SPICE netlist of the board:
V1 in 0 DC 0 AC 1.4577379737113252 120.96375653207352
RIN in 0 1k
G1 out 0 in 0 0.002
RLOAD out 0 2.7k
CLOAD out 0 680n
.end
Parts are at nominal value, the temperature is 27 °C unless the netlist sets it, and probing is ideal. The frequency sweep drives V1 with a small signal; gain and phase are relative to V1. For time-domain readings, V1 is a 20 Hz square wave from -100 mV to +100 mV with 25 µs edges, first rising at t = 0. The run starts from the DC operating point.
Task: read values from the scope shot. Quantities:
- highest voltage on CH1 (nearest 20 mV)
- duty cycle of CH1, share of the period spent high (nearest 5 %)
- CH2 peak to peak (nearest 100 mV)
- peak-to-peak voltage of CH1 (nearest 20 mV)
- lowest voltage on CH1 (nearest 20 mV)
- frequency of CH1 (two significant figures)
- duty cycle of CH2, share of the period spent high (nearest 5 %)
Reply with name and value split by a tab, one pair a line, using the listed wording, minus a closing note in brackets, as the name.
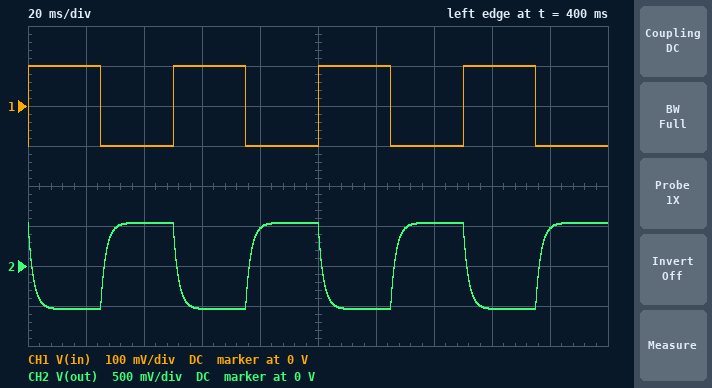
highest voltage on CH1	100 mV
duty cycle of CH1, share of the period spent high	50 %
CH2 peak to peak	1.1 V
peak-to-peak voltage of CH1	200 mV
lowest voltage on CH1	-100 mV
frequency of CH1	20 Hz
duty cycle of CH2, share of the period spent high	50 %
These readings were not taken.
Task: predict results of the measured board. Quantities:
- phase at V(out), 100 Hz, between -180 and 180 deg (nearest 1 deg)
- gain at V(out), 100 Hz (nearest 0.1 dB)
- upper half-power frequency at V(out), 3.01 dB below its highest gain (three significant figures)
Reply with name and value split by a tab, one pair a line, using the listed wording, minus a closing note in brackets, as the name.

phase at V(out), 100 Hz, between -180 and 180 deg	131 deg
gain at V(out), 100 Hz	11.0 dB
upper half-power frequency at V(out), 3.01 dB below its highest gain	86.7 Hz
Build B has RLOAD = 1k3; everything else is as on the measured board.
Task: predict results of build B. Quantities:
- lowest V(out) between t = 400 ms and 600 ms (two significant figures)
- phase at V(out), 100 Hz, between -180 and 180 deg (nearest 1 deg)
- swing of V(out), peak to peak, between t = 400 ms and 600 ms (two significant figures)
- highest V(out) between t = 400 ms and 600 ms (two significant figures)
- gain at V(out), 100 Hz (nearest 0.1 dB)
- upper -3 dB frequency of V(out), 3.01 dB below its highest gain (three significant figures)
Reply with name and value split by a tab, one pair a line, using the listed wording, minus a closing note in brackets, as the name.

lowest V(out) between t = 400 ms and 600 ms	-260 mV
phase at V(out), 100 Hz, between -180 and 180 deg	151 deg
swing of V(out), peak to peak, between t = 400 ms and 600 ms	520 mV
highest V(out) between t = 400 ms and 600 ms	260 mV
gain at V(out), 100 Hz	7.1 dB
upper -3 dB frequency of V(out), 3.01 dB below its highest gain	180 Hz
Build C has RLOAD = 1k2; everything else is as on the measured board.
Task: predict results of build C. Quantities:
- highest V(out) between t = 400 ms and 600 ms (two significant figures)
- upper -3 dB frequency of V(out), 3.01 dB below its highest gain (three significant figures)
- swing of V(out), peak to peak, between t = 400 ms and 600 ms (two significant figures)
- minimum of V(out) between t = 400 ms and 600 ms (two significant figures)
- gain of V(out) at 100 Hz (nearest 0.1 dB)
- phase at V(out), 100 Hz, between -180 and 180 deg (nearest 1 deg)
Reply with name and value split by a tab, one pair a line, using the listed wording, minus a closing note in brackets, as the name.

highest V(out) between t = 400 ms and 600 ms	240 mV
upper -3 dB frequency of V(out), 3.01 dB below its highest gain	195 Hz
swing of V(out), peak to peak, between t = 400 ms and 600 ms	480 mV
minimum of V(out) between t = 400 ms and 600 ms	-240 mV
gain of V(out) at 100 Hz	6.6 dB
phase at V(out), 100 Hz, between -180 and 180 deg	153 deg
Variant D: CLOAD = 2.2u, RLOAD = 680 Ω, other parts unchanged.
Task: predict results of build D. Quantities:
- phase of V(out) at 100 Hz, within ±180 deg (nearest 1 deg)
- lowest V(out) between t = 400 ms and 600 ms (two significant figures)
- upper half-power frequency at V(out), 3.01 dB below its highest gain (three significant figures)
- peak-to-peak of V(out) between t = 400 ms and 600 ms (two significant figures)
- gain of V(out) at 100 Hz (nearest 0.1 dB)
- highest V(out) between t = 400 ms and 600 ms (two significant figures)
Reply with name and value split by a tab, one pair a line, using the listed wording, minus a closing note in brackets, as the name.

phase of V(out) at 100 Hz, within ±180 deg	137 deg
lowest V(out) between t = 400 ms and 600 ms	-140 mV
upper half-power frequency at V(out), 3.01 dB below its highest gain	106 Hz
peak-to-peak of V(out) between t = 400 ms and 600 ms	270 mV
gain of V(out) at 100 Hz	-0.1 dB
highest V(out) between t = 400 ms and 600 ms	140 mV
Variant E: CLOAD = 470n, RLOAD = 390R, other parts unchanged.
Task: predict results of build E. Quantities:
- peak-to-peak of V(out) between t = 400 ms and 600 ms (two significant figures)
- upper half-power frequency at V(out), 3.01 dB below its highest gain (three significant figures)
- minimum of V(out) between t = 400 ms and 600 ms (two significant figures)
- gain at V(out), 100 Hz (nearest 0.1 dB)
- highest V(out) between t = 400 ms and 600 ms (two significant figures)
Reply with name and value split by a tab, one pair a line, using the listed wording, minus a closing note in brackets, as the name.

peak-to-peak of V(out) between t = 400 ms and 600 ms	160 mV
upper half-power frequency at V(out), 3.01 dB below its highest gain	868 Hz
minimum of V(out) between t = 400 ms and 600 ms	-78 mV
gain at V(out), 100 Hz	-2.2 dB
highest V(out) between t = 400 ms and 600 ms	78 mV
